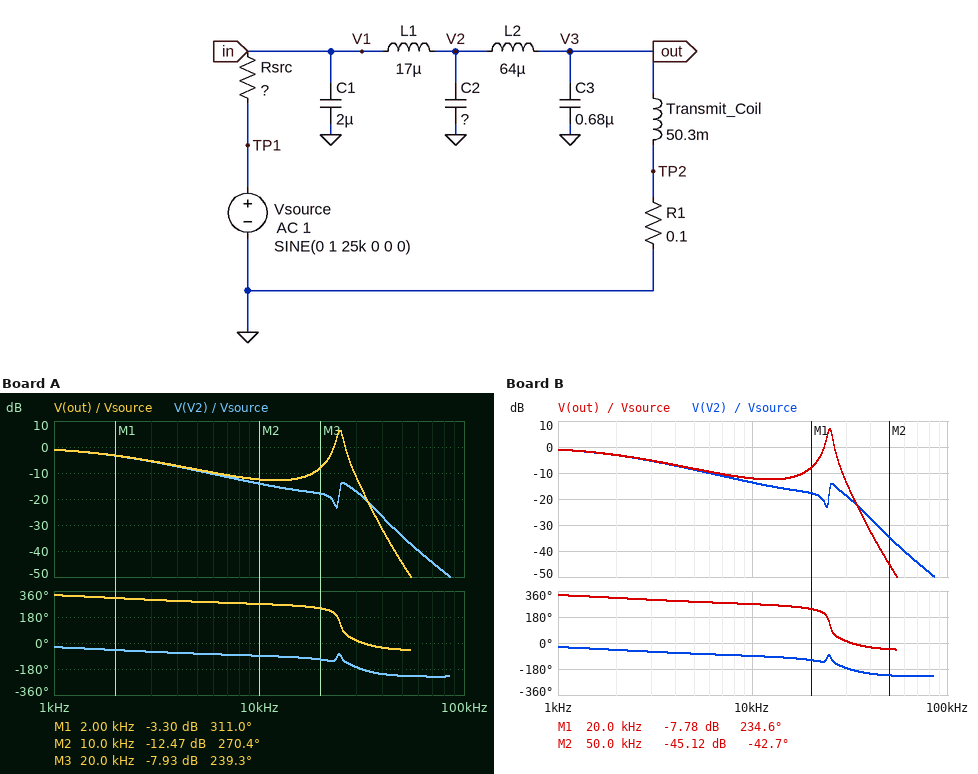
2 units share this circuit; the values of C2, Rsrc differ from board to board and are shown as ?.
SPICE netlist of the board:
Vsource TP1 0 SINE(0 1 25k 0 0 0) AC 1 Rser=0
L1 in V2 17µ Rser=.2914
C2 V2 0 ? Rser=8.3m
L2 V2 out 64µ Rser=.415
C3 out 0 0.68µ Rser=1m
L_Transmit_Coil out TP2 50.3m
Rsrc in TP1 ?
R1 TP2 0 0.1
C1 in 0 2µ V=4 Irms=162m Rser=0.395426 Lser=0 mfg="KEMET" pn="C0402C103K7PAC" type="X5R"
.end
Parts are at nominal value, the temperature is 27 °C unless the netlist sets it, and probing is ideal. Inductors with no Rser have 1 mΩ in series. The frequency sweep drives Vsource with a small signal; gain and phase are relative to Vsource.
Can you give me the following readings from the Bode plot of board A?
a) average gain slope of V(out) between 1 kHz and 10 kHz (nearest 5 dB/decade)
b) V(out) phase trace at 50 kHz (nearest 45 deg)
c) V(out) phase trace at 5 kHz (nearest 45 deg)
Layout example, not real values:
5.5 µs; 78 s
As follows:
-10 dB/decade; -45 deg; 270 deg
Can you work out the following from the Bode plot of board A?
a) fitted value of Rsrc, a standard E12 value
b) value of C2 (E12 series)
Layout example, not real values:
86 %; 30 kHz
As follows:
6.8 Ω; 10 µF
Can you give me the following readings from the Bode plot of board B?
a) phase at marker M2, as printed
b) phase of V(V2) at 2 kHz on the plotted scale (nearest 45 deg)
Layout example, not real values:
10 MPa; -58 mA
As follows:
-42.7 deg; -45 deg
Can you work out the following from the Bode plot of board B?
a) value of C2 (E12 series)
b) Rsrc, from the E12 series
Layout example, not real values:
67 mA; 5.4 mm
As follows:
12 µF; 5.6 Ω
